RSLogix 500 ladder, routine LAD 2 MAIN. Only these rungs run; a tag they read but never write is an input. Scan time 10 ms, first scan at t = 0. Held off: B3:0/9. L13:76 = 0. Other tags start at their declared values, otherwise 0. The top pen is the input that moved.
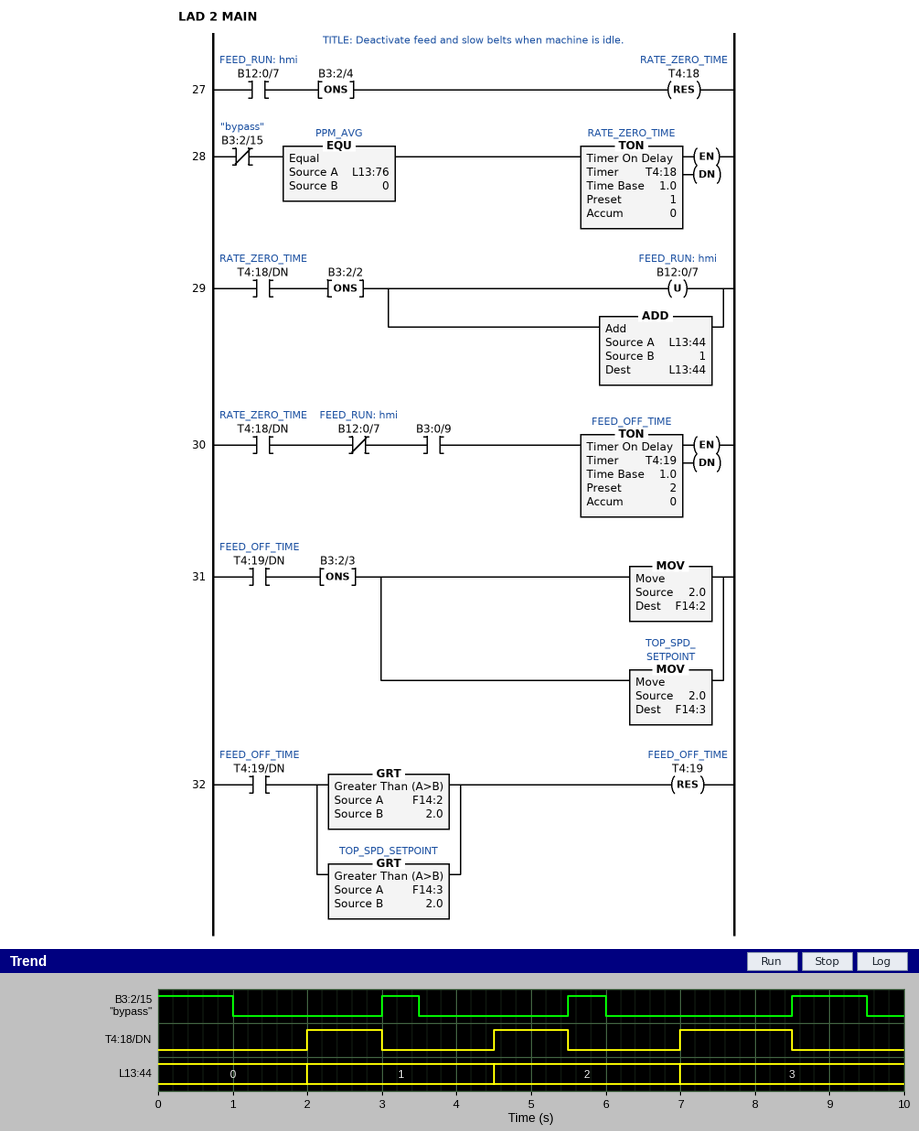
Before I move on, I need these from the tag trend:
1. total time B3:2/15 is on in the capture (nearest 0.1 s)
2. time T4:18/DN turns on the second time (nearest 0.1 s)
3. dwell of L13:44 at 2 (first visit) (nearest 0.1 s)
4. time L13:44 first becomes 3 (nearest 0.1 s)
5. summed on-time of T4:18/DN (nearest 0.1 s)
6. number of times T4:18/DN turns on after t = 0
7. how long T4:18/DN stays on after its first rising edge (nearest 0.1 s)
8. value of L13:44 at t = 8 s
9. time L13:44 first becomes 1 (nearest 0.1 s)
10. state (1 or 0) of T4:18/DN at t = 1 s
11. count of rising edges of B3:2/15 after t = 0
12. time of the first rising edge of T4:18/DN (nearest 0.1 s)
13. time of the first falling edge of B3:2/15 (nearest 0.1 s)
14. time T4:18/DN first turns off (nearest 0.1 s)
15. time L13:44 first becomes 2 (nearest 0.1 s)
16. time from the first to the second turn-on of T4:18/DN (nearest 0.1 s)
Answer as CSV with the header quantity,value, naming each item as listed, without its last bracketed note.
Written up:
quantity,value
total time B3:2/15 is on in the capture,3.0 s
time T4:18/DN turns on the second time,4.5 s
dwell of L13:44 at 2 (first visit),2.5 s
time L13:44 first becomes 3,7.0 s
summed on-time of T4:18/DN,3.5 s
number of times T4:18/DN turns on after t = 0,3
how long T4:18/DN stays on after its first rising edge,1.0 s
value of L13:44 at t = 8 s,3
time L13:44 first becomes 1,2.0 s
state (1 or 0) of T4:18/DN at t = 1 s,0
count of rising edges of B3:2/15 after t = 0,3
time of the first rising edge of T4:18/DN,2.0 s
time of the first falling edge of B3:2/15,1.0 s
time T4:18/DN first turns off,3.0 s
time L13:44 first becomes 2,4.5 s
time from the first to the second turn-on of T4:18/DN,2.5 s
